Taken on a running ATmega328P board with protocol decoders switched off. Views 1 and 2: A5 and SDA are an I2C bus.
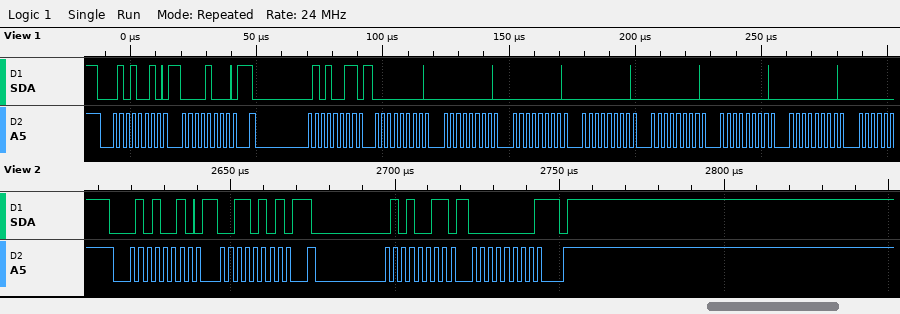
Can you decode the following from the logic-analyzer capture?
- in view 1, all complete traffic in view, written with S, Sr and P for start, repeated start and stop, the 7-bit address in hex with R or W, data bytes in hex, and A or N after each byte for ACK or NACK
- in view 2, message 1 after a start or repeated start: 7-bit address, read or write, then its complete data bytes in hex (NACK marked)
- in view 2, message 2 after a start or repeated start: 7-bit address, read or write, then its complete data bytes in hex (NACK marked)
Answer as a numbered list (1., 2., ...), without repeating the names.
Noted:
1. S 29W A 08 A Sr 29R A 00 A 00 A 00 A 00 A 00 A 00 A 00 A
2. 0x29 write: 35
3. 0x29 read: 00 NACK
